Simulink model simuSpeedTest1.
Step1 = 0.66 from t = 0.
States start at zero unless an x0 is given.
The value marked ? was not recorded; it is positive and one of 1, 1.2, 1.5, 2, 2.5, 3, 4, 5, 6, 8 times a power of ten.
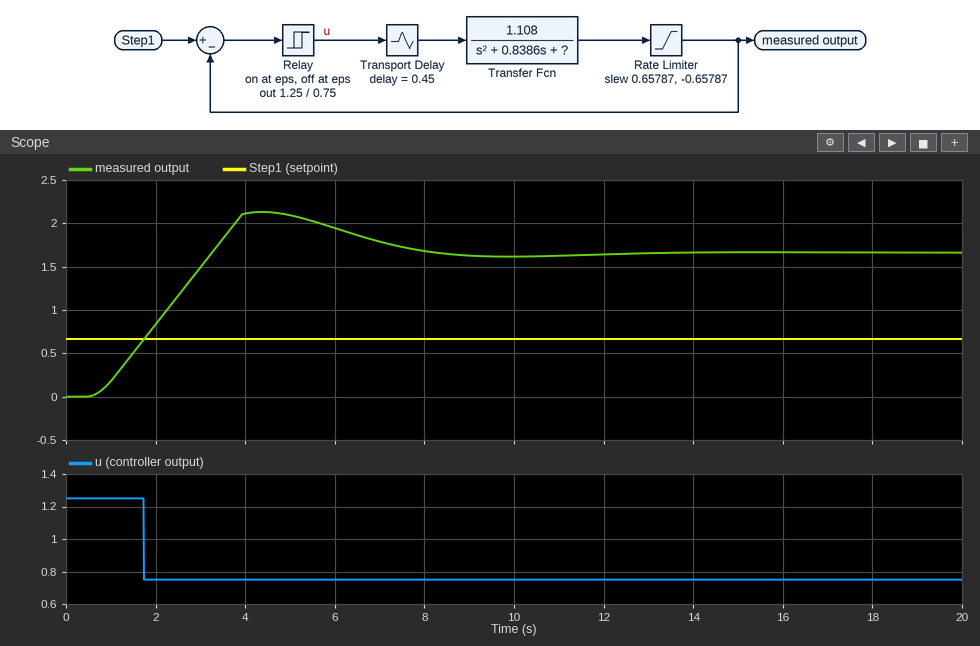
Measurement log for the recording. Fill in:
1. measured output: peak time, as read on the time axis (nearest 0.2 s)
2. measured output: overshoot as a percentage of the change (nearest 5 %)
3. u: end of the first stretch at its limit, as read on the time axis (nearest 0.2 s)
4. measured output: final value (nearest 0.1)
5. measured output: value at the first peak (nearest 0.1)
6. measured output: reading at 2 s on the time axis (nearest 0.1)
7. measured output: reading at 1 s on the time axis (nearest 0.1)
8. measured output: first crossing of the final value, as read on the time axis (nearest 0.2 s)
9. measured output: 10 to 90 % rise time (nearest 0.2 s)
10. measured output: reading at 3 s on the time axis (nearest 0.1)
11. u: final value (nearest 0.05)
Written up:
4.4 s
30 %
1.8 s
1.7
2.1
0.8
0.2
3.2 s
2.0 s
1.5
0.75
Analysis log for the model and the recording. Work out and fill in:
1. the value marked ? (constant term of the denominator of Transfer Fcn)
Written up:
0.5
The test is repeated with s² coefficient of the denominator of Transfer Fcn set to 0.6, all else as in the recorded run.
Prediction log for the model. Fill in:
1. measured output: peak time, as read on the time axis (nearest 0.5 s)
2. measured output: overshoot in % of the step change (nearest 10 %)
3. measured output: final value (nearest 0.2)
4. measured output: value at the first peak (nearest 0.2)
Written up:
3.5 s
20 %
1.6
2.0
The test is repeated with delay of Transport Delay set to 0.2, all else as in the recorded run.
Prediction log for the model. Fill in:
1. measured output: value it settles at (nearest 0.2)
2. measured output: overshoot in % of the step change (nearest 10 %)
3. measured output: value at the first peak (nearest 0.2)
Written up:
1.6
20 %
2.0
